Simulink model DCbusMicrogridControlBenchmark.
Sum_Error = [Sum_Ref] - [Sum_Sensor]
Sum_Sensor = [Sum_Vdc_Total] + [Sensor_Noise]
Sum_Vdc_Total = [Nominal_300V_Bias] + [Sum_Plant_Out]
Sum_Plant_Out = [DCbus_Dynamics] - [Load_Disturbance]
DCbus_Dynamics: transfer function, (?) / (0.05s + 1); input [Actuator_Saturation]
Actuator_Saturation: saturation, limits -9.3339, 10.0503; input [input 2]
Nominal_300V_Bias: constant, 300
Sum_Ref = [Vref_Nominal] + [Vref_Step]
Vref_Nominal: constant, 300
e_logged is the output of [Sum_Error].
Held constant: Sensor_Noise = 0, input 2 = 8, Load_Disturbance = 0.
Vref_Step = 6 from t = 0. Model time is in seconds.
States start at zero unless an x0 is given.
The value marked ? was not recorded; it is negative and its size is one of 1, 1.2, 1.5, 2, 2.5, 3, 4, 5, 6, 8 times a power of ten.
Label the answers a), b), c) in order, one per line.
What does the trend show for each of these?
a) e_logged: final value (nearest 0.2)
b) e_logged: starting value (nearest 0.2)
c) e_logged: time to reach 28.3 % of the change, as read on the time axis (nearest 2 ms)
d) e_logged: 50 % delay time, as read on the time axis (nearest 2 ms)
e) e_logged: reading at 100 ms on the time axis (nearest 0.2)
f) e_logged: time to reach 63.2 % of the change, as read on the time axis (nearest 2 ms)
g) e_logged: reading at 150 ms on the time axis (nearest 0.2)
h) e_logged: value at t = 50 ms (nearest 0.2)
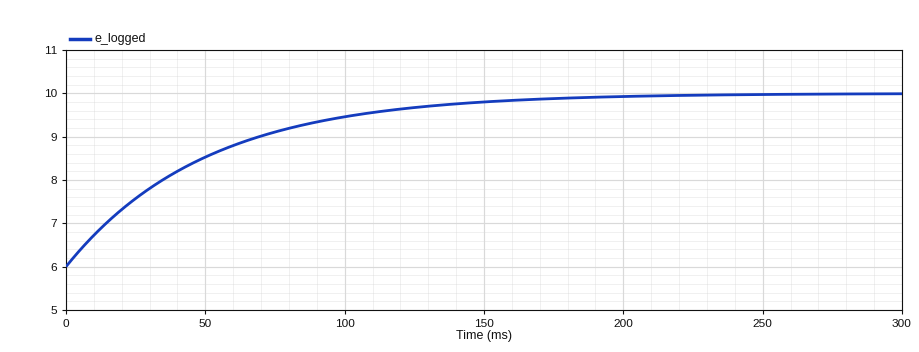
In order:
a) 10.0
b) 6.0
c) 16 ms
d) 34 ms
e) 9.4
f) 50 ms
g) 9.8
h) 8.6
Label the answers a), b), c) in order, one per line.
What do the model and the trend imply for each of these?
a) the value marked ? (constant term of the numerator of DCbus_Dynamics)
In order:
a) -0.5
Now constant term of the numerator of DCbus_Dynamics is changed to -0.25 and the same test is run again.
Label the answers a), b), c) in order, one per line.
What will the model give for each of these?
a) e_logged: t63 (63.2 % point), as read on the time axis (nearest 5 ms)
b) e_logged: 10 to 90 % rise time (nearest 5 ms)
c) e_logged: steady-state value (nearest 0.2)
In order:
a) 50 ms
b) 110 ms
c) 8.0
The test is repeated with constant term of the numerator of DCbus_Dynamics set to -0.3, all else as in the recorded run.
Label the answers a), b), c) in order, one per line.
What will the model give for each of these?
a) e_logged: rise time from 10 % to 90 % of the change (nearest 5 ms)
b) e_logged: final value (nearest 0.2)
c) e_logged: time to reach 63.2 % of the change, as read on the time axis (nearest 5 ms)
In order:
a) 110 ms
b) 8.4
c) 50 ms
